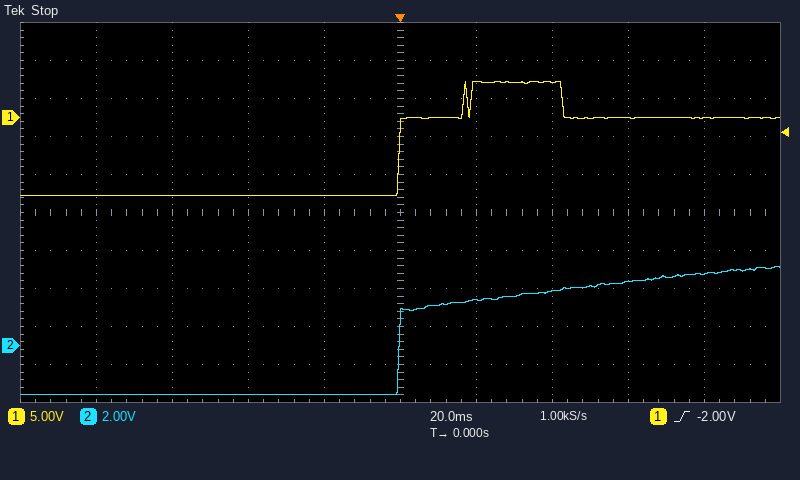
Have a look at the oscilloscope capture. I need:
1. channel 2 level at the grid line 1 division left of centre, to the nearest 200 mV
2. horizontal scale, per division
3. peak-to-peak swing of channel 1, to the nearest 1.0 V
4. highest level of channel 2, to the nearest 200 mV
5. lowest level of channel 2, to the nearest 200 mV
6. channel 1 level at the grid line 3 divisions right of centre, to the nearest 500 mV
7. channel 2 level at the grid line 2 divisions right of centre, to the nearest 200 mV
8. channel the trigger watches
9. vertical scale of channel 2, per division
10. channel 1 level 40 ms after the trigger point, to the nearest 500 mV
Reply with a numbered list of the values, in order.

1. -2.6 V
2. 20 ms
3. 15.0 V
4. 4.2 V
5. -2.6 V
6. 0.0 V
7. 2.8 V
8. channel 1
9. 2 V
10. 4.5 V
